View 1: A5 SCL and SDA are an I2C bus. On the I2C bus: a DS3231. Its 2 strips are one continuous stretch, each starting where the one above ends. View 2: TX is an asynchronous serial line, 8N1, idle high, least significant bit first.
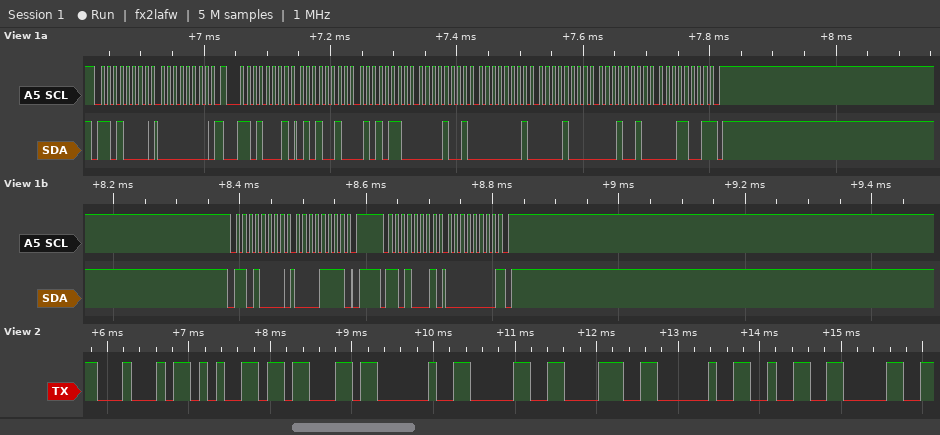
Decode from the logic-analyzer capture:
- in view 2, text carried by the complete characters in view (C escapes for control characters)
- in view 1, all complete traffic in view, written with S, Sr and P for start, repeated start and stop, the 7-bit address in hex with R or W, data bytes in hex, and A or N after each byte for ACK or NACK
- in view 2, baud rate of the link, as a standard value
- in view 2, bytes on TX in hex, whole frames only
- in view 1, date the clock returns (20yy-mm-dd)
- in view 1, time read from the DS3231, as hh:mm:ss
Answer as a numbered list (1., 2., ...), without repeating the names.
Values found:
1. "Dec 08 20"
2. S 68W A 00 A Sr 68R A 52 A 56 A 09 A 01 A 08 A 12 A 19 N P S 68W A 0F A P S 68R A 00 N P
3. 9600 baud
4. 44 65 63 20 30 38 20 32 30
5. 2019-12-08
6. 09:56:52
